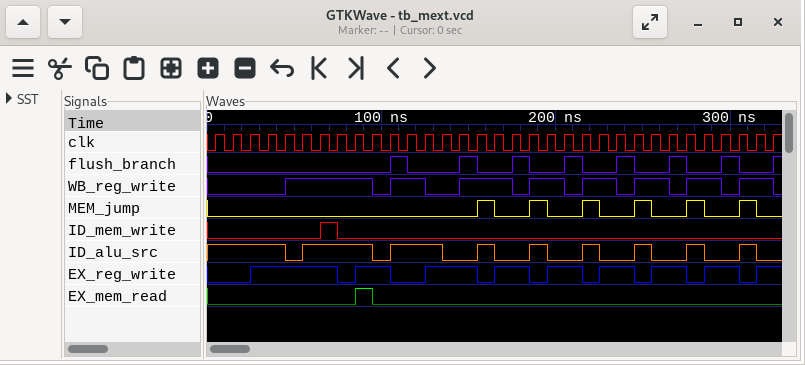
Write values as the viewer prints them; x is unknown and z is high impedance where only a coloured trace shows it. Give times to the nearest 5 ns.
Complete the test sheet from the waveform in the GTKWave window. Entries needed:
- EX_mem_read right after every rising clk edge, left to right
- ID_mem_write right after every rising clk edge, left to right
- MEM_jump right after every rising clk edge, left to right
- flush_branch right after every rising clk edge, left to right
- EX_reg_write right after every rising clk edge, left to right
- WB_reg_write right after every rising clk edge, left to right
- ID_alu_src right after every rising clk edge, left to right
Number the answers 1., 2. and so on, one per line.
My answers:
1. 0 0 0 0 0 0 0 0 1 0 0 0 0 0 0 0 0 0 0 0 0 0 0 0 0 0 0 0 0 0 0 0 0
2. 0 0 0 0 0 0 1 0 0 0 0 0 0 0 0 0 0 0 0 0 0 0 0 0 0 0 0 0 0 0 0 0 0
3. 0 0 0 0 0 0 0 0 0 0 0 0 0 0 0 1 0 0 1 0 0 1 0 0 1 0 0 1 0 0 1 0 0
4. 0 0 0 0 0 0 0 0 0 0 1 0 0 0 1 0 0 1 0 0 1 0 0 1 0 0 1 0 0 1 0 0 1
5. 0 0 1 1 1 1 1 0 1 1 0 0 1 1 1 0 1 1 0 1 1 0 1 1 0 1 1 0 1 1 0 1 1
6. 0 0 0 0 1 1 1 1 1 0 1 1 0 0 1 1 1 0 1 1 0 1 1 0 1 1 0 1 1 0 1 1 0
7. 1 1 1 1 0 1 1 1 1 0 1 1 1 0 0 1 0 0 1 0 0 1 0 0 1 0 0 1 0 0 1 0 0
